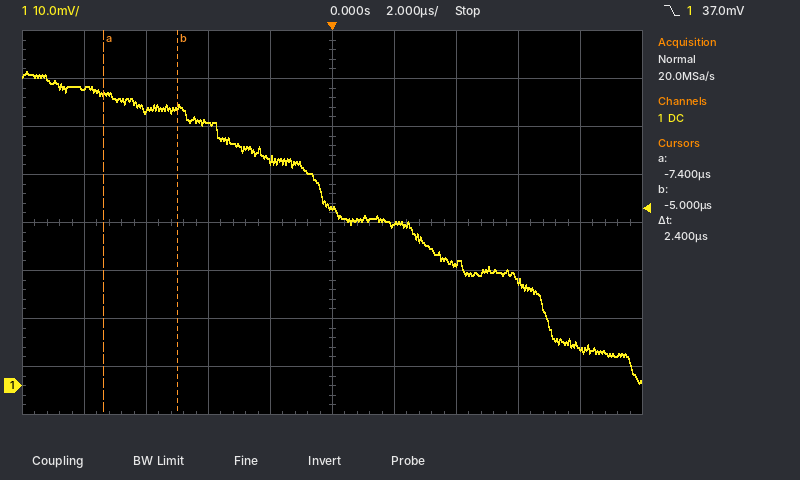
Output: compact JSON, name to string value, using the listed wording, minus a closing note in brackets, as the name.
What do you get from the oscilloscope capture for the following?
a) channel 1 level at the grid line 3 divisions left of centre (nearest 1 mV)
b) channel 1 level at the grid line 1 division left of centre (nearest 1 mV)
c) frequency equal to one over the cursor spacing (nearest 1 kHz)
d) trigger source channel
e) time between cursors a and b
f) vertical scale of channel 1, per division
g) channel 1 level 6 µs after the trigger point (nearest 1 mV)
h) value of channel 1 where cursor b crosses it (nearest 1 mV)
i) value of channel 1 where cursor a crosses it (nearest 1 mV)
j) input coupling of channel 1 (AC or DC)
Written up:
{"channel 1 level at the grid line 3 divisions left of centre": "57 mV", "channel 1 level at the grid line 1 division left of centre": "47 mV", "frequency equal to one over the cursor spacing": "417 kHz", "trigger source channel": "channel 1", "time between cursors a and b": "2.4 µs", "vertical scale of channel 1, per division": "10 mV", "channel 1 level 6 µs after the trigger point": "22 mV", "value of channel 1 where cursor b crosses it": "58 mV", "value of channel 1 where cursor a crosses it": "61 mV", "input coupling of channel 1": "DC"}
